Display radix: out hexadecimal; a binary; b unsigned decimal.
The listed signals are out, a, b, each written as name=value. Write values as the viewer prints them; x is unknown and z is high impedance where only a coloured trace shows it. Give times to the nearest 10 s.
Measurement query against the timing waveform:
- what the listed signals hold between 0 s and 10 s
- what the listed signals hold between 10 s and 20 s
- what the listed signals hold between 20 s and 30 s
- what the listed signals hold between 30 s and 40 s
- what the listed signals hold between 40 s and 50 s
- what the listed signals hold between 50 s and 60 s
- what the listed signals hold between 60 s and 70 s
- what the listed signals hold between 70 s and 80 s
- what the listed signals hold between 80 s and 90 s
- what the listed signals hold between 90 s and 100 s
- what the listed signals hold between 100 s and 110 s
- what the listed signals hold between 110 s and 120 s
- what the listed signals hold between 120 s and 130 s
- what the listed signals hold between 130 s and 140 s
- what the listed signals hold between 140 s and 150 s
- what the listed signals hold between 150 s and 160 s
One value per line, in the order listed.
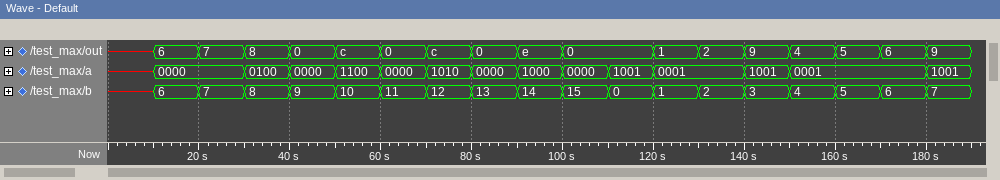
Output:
out=x, a=x, b=x
out=6, a=0000, b=6
out=7, a=0000, b=7
out=8, a=0100, b=8
out=0, a=0000, b=9
out=c, a=1100, b=10
out=0, a=0000, b=11
out=c, a=1010, b=12
out=0, a=0000, b=13
out=e, a=1000, b=14
out=0, a=0000, b=15
out=0, a=1001, b=0
out=1, a=0001, b=1
out=2, a=0001, b=2
out=9, a=1001, b=3
out=4, a=0001, b=4
